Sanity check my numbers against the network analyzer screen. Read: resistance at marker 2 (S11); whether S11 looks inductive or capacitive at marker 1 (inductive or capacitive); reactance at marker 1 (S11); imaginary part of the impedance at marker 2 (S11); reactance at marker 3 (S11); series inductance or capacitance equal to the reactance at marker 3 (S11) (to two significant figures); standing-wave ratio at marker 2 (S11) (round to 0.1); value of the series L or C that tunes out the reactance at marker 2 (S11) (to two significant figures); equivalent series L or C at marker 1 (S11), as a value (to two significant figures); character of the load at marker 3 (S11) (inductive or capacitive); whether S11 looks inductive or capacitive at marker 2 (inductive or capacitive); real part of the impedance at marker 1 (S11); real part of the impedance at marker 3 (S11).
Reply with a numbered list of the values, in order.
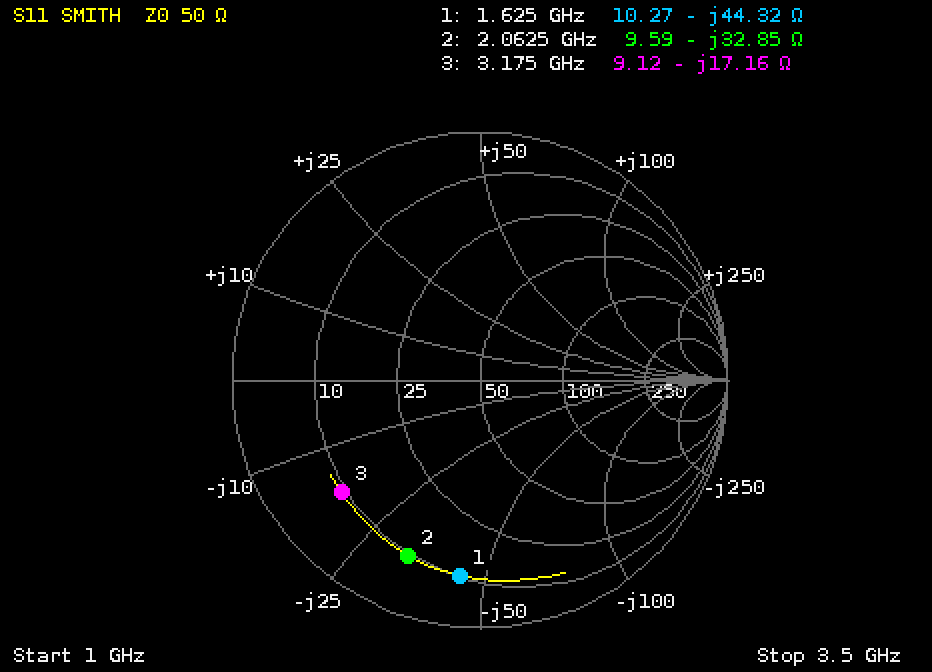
1. 9.59 Ω
2. capacitive
3. -44.32 Ω
4. -32.85 Ω
5. -17.16 Ω
6. 2.9 pF
7. 7.5
8. 2.5 nH
9. 2.2 pF
10. capacitive
11. capacitive
12. 10.27 Ω
13. 9.12 Ω
